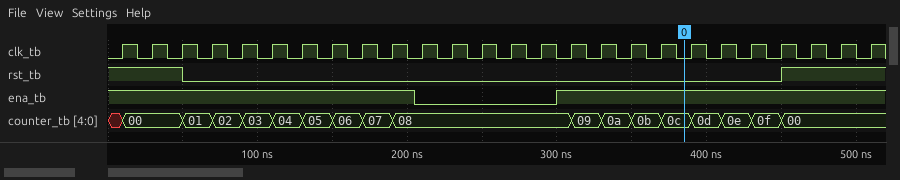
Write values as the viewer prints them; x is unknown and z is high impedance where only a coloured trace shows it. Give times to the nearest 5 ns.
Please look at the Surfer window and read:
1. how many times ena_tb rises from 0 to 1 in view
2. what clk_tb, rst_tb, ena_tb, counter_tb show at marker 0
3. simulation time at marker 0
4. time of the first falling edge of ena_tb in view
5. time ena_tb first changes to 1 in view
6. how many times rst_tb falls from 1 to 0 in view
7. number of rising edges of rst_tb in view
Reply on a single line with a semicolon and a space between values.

1; clk_tb=0, rst_tb=0, ena_tb=1, counter_tb=0c; 385 ns; 205 ns; 300 ns; 1; 1
